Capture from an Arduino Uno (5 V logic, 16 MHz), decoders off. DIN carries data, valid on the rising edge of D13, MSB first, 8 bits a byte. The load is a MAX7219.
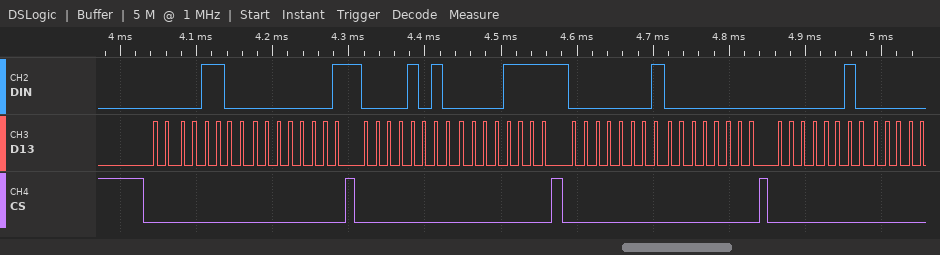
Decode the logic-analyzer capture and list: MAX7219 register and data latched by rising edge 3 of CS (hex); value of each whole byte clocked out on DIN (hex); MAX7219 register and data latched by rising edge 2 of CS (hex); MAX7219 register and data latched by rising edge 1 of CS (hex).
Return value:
register 0x1, data 0x00
0x0C 0x01 0x0A 0x0F 0x01 0x00 0x02
register 0xA, data 0x0F
register 0xC, data 0x01
